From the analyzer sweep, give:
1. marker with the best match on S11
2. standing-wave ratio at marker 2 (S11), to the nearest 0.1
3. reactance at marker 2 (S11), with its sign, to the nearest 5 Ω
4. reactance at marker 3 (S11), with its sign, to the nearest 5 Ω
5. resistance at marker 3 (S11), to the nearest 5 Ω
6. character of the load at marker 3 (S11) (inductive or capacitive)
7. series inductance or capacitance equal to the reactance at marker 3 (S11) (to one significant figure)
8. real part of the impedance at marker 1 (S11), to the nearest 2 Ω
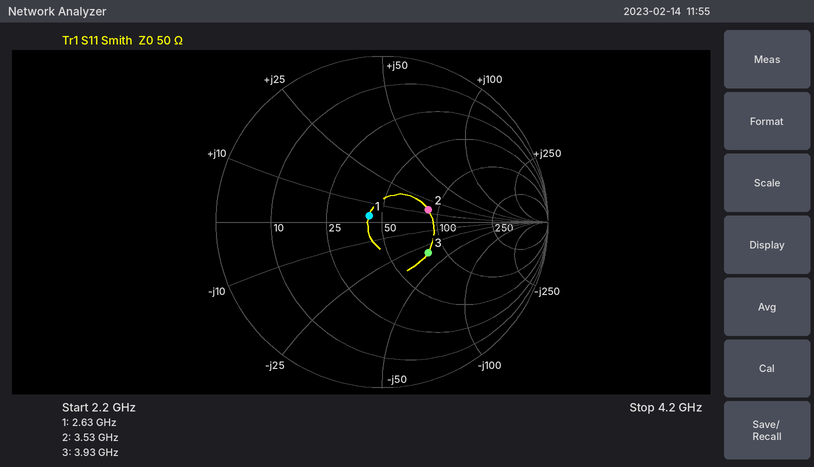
marker 1
1.8
+15 Ω
-35 Ω
80 Ω
capacitive
1 pF
42 Ω
